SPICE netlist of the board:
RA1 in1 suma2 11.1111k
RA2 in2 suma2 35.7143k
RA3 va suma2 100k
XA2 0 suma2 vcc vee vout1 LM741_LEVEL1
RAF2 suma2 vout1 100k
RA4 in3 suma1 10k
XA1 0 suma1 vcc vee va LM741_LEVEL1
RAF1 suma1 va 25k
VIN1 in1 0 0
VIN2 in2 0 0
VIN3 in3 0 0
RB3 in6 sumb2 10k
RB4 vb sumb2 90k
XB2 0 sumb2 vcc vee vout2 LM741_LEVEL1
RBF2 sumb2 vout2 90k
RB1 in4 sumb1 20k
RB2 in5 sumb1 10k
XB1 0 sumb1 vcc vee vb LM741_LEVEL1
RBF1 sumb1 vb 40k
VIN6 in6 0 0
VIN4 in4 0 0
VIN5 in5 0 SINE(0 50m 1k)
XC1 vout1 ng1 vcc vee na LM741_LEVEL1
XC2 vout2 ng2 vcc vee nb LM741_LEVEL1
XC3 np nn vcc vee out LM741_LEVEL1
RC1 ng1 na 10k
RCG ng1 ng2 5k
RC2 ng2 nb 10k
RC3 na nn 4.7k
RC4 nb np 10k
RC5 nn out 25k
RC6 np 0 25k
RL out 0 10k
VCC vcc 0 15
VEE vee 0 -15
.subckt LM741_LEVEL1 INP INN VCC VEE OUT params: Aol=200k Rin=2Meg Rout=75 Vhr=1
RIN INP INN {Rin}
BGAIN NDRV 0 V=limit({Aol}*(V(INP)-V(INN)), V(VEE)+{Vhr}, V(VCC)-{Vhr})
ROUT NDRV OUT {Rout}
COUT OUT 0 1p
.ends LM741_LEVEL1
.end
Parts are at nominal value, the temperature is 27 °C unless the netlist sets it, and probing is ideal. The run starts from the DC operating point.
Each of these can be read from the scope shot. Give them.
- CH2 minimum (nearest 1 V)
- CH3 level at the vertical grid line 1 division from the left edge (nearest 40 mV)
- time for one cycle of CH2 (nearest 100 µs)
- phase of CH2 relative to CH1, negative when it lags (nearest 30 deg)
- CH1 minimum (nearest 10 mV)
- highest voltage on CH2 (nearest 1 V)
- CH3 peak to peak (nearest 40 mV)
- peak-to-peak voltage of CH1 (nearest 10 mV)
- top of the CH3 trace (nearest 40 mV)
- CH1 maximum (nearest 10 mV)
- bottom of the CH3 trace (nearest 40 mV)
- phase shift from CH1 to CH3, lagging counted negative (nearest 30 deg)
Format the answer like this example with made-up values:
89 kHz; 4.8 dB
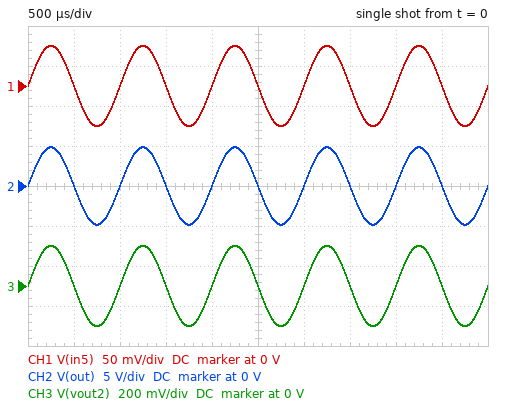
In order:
-5 V; 0 V; 1.0 ms; 0 deg; -50 mV; 5 V; 400 mV; 100 mV; 200 mV; 50 mV; -200 mV; 0 deg
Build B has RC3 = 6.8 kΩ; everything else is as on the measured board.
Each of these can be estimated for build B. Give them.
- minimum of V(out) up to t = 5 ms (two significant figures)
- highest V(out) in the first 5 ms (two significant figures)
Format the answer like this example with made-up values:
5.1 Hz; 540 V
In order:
-3.5 V; 3.5 V
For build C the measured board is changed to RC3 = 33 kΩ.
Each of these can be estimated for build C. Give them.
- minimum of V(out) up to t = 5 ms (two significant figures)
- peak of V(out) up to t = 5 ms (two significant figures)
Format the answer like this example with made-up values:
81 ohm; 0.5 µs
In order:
-1.1 V; 1.1 V
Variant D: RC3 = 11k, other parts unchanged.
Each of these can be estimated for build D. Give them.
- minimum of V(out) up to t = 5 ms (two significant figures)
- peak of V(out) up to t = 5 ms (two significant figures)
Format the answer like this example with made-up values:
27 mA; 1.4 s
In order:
-2.3 V; 2.3 V
